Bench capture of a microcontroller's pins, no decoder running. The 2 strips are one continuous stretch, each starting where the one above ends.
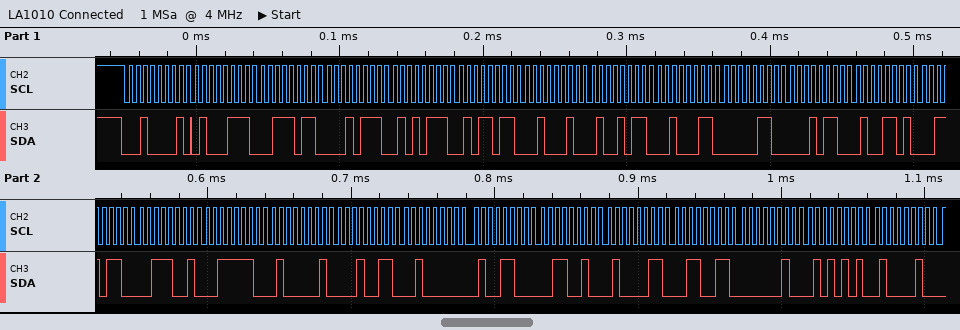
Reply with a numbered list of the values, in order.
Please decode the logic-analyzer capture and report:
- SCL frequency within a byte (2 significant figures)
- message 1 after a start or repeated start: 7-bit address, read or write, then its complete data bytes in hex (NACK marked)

1. 200 kHz
2. 0x10 read: 47 3B 17 57 5B 22 4B 23 06 16 4D 36 39 3E 41 13 20 4C 32 43 33 02 55 42
